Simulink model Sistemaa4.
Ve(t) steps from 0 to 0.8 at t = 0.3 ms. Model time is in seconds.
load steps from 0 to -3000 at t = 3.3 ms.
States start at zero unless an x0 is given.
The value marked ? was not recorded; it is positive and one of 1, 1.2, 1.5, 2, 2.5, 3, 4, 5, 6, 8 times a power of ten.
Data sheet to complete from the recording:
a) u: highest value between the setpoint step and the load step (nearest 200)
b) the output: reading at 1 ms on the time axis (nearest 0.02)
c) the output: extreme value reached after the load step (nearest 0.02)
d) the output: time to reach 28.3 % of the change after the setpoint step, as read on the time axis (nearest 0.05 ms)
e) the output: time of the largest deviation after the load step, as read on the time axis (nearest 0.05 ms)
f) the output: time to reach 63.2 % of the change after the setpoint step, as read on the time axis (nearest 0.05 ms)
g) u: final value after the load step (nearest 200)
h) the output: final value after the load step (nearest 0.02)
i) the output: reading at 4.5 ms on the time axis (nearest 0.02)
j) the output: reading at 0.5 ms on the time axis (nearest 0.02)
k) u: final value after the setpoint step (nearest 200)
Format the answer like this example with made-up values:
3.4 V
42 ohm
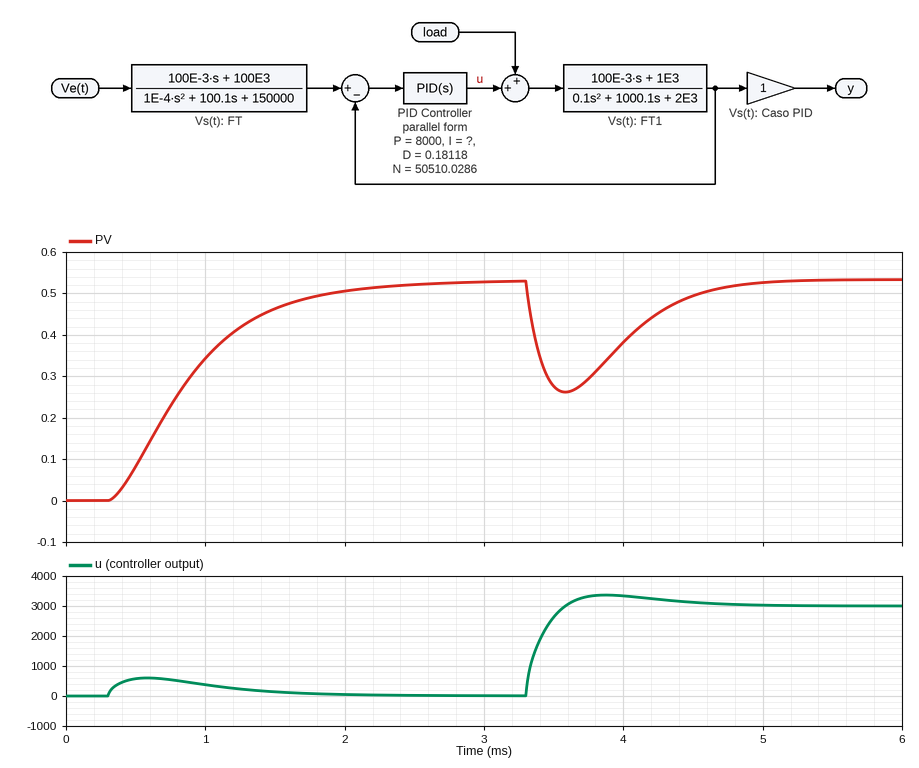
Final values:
600
0.34
0.26
0.60 ms
3.60 ms
1.00 ms
3000
0.54
0.50
0.08
0
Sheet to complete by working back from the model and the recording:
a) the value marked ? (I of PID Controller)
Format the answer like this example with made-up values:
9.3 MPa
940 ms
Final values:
1.5e+07
